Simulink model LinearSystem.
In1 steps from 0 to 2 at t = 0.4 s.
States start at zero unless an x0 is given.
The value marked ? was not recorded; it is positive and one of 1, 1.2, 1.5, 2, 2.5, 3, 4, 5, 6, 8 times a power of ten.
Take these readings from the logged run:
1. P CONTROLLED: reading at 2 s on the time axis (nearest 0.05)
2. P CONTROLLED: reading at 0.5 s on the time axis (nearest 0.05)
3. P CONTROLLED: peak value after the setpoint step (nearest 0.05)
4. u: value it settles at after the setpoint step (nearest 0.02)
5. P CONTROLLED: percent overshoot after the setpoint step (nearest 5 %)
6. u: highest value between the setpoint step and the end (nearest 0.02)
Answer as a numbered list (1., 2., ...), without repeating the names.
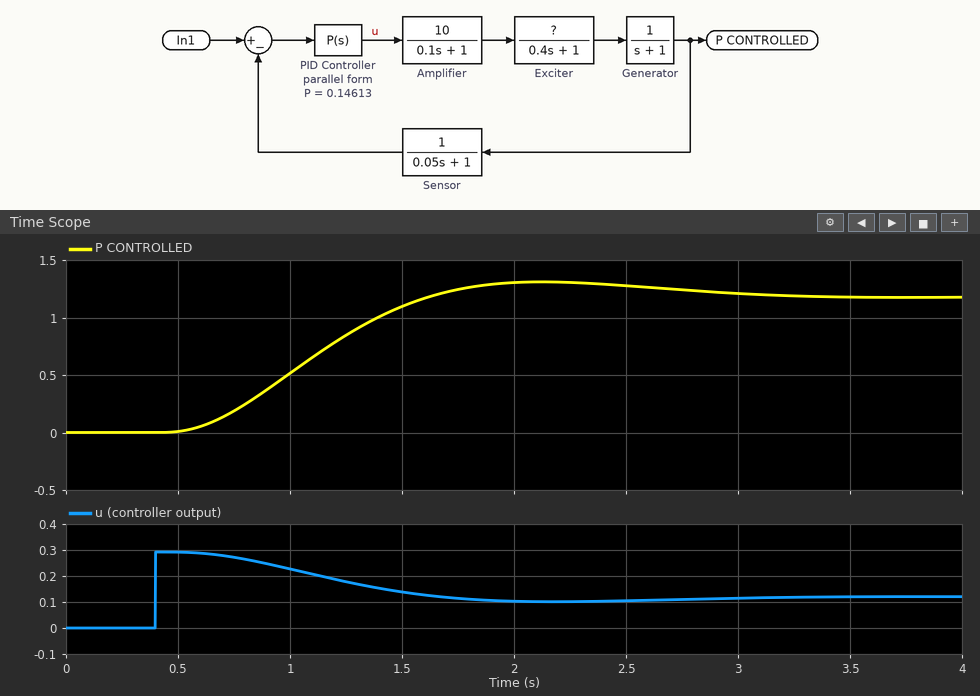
1. 1.30
2. 0.00
3. 1.30
4. 0.12
5. 10 %
6. 0.30
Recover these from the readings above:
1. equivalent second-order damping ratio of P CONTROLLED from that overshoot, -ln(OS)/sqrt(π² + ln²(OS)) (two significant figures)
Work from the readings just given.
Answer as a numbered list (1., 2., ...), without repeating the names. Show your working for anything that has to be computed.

1. ln(0.1) = -2.303; 2.303 / sqrt(9.870 + 5.302) = 0.59
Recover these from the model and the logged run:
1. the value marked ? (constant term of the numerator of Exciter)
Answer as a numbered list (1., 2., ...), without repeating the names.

1. 1
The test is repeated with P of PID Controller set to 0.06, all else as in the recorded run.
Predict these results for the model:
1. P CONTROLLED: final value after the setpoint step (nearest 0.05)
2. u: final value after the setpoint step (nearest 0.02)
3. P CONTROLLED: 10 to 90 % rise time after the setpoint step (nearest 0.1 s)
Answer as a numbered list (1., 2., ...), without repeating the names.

1. 0.75
2. 0.08
3. 1.3 s
